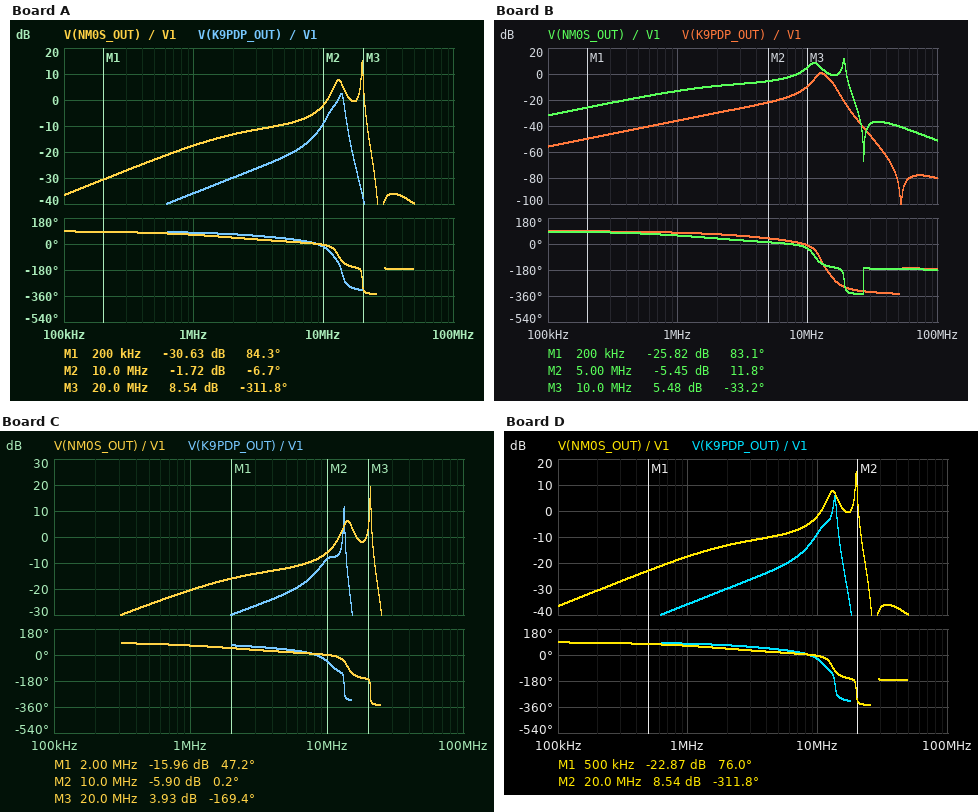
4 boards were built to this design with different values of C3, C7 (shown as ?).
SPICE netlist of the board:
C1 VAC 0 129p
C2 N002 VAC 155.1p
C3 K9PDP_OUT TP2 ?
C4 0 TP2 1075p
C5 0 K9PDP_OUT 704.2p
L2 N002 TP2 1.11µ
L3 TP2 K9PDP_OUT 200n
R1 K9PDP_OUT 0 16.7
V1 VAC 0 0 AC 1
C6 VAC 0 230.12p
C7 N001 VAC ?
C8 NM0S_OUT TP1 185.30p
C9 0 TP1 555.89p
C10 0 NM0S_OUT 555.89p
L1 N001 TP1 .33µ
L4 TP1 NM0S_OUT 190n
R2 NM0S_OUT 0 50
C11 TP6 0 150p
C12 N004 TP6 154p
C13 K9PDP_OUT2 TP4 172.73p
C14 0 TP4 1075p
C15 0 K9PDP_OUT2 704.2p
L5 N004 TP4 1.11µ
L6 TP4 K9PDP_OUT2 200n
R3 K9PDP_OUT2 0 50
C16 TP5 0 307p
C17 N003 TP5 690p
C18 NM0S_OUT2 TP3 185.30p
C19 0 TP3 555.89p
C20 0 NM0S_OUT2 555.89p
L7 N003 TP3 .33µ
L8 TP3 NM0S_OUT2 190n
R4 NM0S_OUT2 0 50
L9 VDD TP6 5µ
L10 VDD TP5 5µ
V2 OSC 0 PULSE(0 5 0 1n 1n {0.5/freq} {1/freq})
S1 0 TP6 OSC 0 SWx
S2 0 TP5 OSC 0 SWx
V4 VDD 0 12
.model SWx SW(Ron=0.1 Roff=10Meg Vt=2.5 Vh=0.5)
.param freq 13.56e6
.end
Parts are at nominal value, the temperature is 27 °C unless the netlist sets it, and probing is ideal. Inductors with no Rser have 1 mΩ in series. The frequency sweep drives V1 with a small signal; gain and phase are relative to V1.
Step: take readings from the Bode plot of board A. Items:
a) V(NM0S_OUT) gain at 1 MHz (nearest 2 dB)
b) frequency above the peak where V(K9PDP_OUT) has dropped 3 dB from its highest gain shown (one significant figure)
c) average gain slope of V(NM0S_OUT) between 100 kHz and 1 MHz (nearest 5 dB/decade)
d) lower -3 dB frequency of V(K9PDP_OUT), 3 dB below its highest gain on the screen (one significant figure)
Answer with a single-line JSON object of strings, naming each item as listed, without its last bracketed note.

{"V(NM0S_OUT) gain at 1 MHz": "-18 dB", "frequency above the peak where V(K9PDP_OUT) has dropped 3 dB from its highest gain shown": "10 MHz", "average gain slope of V(NM0S_OUT) between 100 kHz and 1 MHz": "20 dB/decade", "lower -3 dB frequency of V(K9PDP_OUT), 3 dB below its highest gain on the screen": "10 MHz"}
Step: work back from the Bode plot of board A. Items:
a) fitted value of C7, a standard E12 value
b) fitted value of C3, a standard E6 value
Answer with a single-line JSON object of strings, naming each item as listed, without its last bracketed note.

{"fitted value of C7, a standard E12 value": "470 pF", "fitted value of C3, a standard E6 value": "220 pF"}
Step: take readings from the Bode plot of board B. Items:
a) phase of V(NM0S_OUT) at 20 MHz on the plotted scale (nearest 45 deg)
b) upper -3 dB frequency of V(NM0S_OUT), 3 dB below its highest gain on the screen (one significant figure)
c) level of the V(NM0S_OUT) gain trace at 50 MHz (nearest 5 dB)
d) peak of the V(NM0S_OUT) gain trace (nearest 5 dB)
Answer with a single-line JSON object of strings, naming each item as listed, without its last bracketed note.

{"phase of V(NM0S_OUT) at 20 MHz on the plotted scale": "-315 deg", "upper -3 dB frequency of V(NM0S_OUT), 3 dB below its highest gain on the screen": "20 MHz", "level of the V(NM0S_OUT) gain trace at 50 MHz": "-40 dB", "peak of the V(NM0S_OUT) gain trace": "10 dB"}
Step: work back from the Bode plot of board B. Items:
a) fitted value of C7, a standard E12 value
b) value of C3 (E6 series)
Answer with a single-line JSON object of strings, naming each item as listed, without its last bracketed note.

{"fitted value of C7, a standard E12 value": "820 pF", "value of C3": "47 pF"}
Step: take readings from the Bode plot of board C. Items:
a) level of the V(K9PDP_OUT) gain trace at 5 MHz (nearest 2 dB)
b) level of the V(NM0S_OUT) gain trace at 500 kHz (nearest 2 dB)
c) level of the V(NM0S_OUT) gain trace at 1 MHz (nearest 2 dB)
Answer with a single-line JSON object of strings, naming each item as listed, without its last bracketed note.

{"level of the V(K9PDP_OUT) gain trace at 5 MHz": "-22 dB", "level of the V(NM0S_OUT) gain trace at 500 kHz": "-26 dB", "level of the V(NM0S_OUT) gain trace at 1 MHz": "-20 dB"}
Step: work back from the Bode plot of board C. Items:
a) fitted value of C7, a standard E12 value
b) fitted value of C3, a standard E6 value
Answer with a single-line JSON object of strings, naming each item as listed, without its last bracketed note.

{"fitted value of C7, a standard E12 value": "330 pF", "fitted value of C3, a standard E6 value": "470 pF"}
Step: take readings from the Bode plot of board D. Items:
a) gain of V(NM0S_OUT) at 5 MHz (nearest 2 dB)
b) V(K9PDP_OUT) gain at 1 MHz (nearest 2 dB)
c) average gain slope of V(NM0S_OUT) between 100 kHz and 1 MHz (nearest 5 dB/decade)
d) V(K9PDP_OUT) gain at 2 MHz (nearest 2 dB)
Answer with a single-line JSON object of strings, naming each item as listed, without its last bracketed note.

{"gain of V(NM0S_OUT) at 5 MHz": "-10 dB", "V(K9PDP_OUT) gain at 1 MHz": "-36 dB", "average gain slope of V(NM0S_OUT) between 100 kHz and 1 MHz": "20 dB/decade", "V(K9PDP_OUT) gain at 2 MHz": "-30 dB"}
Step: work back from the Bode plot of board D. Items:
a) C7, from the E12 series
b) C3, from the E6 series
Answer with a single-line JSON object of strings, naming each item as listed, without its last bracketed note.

{"C7, from the E12 series": "470 pF", "C3, from the E6 series": "330 pF"}
